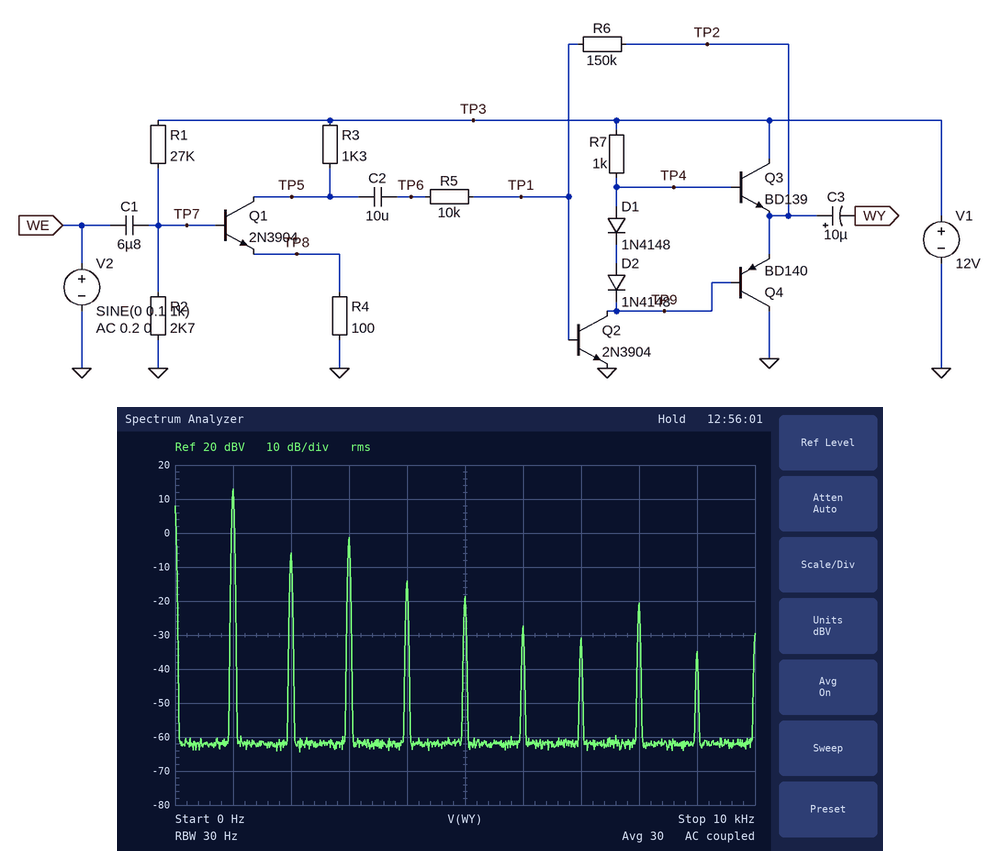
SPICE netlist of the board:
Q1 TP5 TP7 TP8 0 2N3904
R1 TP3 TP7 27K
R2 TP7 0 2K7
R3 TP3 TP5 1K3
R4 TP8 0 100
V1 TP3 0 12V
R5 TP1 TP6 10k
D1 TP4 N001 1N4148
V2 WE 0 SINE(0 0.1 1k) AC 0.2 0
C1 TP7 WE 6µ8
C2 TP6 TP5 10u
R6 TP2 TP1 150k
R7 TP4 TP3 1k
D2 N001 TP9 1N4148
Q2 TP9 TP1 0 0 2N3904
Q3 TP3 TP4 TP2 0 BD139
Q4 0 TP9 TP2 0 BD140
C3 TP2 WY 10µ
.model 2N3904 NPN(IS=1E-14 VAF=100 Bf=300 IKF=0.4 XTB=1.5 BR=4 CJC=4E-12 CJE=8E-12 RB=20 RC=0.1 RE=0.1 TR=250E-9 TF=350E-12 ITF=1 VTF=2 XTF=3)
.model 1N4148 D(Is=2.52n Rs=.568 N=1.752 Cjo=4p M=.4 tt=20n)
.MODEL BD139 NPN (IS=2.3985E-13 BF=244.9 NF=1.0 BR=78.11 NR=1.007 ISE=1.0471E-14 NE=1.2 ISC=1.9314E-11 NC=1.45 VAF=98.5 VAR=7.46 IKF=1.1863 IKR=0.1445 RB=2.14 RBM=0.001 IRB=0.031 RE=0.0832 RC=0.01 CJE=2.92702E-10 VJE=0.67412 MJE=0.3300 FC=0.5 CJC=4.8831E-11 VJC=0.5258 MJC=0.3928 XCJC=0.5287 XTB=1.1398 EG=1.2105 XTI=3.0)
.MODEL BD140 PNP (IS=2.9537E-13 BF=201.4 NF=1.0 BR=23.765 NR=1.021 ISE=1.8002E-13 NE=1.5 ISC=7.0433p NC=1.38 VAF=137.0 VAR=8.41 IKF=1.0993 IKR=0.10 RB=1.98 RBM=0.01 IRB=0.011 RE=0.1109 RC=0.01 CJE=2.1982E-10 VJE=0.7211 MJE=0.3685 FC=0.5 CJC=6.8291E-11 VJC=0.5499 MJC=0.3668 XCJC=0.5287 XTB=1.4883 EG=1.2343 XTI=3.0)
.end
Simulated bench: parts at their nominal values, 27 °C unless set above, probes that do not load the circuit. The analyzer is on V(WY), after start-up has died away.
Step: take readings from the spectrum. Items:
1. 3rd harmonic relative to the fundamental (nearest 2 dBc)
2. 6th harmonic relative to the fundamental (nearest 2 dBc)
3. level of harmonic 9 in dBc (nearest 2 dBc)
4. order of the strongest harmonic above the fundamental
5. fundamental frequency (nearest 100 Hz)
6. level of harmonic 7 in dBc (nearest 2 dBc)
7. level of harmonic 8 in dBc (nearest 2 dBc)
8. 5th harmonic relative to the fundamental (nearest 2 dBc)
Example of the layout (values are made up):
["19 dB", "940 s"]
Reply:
["-14 dBc", "-40 dBc", "-48 dBc", "3", "1.0 kHz", "-44 dBc", "-34 dBc", "-32 dBc"]
